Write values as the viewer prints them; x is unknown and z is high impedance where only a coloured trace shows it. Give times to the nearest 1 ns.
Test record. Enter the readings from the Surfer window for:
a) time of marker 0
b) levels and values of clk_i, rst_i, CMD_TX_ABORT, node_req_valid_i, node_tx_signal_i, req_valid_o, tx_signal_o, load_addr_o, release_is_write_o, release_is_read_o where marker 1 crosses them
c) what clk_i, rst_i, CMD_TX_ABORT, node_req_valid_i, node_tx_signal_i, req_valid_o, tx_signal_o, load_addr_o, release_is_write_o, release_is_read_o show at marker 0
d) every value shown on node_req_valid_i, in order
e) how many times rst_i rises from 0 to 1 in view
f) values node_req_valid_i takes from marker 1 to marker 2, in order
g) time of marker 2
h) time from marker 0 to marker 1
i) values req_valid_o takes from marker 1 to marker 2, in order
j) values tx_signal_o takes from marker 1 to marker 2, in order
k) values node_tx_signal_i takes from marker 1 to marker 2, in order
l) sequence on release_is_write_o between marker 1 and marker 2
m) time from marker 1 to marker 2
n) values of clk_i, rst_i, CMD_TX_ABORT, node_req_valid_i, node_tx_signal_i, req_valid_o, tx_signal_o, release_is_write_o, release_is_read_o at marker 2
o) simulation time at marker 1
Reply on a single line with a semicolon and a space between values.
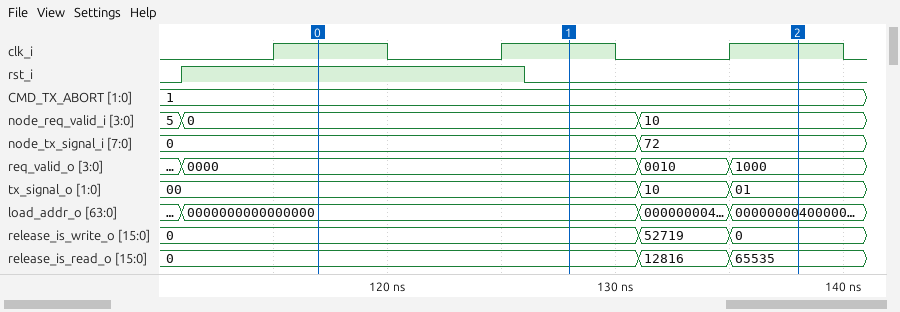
117 ns; clk_i=1, rst_i=0, CMD_TX_ABORT=1, node_req_valid_i=0, node_tx_signal_i=0, req_valid_o=0000, tx_signal_o=00, load_addr_o=0000000000000000, release_is_write_o=0, release_is_read_o=0; clk_i=1, rst_i=1, CMD_TX_ABORT=1, node_req_valid_i=0, node_tx_signal_i=0, req_valid_o=0000, tx_signal_o=00, load_addr_o=0000000000000000, release_is_write_o=0, release_is_read_o=0; 5, 0, 10; 1; 0, 10; 138 ns; 11 ns; 0000, 0010, 1000; 00, 10, 01; 0, 72; 0, 52719, 0; 10 ns; clk_i=1, rst_i=0, CMD_TX_ABORT=1, node_req_valid_i=10, node_tx_signal_i=72, req_valid_o=1000, tx_signal_o=01, release_is_write_o=0, release_is_read_o=65535; 128 ns
